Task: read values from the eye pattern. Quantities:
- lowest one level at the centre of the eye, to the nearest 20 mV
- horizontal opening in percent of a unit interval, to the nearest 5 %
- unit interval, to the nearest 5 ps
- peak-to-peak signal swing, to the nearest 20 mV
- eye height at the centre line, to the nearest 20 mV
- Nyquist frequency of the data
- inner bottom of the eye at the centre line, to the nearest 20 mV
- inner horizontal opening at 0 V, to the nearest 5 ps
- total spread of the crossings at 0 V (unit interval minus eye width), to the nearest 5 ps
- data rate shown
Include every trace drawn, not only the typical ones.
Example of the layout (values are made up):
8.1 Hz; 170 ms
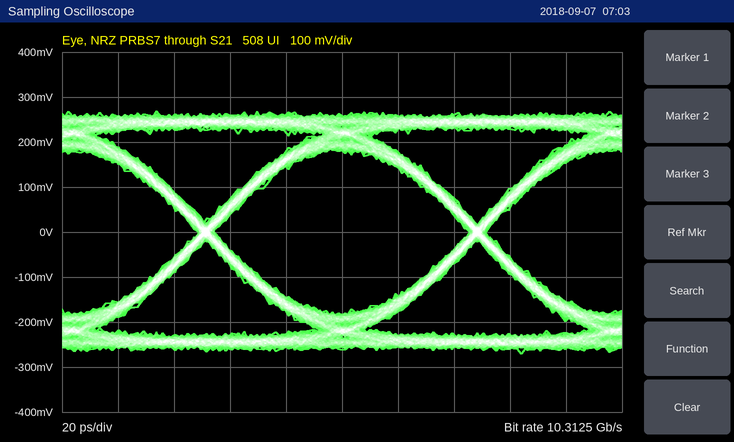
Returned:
180 mV; 95 %; 95 ps; 540 mV; 360 mV; 5.15625 GHz; -180 mV; 90 ps; 5 ps; 10.3125 Gb/s
